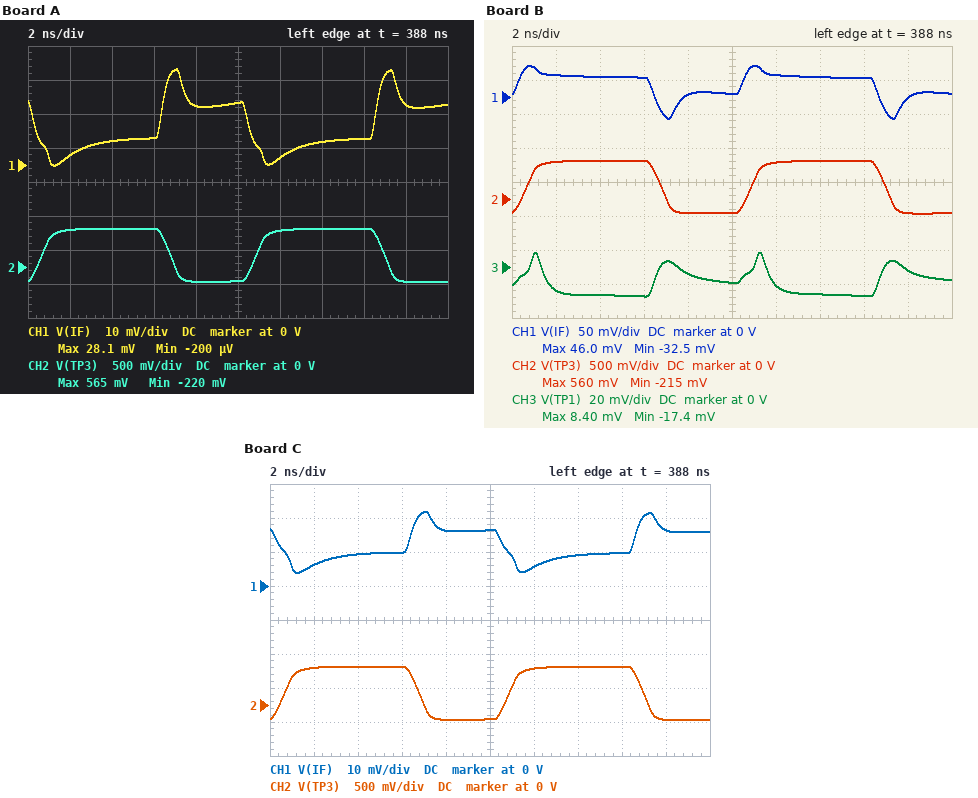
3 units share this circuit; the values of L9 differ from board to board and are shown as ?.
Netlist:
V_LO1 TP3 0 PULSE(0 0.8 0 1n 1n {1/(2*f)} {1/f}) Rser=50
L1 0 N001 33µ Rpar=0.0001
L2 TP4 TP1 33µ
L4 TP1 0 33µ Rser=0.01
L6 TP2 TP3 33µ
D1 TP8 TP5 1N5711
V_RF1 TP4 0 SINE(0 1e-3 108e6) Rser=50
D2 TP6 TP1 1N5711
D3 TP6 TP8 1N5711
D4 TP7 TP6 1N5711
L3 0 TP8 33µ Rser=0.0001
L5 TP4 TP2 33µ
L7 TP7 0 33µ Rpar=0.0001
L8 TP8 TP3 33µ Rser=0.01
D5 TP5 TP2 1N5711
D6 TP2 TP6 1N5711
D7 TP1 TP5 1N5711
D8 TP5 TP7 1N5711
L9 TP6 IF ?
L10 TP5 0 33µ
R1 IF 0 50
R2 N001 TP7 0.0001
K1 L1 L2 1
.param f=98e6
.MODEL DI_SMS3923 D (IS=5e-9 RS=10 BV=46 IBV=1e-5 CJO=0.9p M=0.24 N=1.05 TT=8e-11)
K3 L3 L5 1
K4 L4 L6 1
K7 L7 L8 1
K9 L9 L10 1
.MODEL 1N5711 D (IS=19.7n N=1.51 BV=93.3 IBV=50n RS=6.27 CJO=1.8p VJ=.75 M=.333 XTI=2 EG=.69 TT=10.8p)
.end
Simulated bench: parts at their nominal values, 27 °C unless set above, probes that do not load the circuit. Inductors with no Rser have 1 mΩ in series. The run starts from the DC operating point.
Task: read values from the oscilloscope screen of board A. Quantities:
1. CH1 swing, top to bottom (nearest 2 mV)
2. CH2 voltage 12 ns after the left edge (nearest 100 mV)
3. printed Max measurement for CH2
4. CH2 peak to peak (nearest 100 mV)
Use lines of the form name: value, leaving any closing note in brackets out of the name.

CH1 swing, top to bottom: 28 mV
CH2 voltage 12 ns after the left edge: 500 mV
printed Max measurement for CH2: 565 mV
CH2 peak to peak: 800 mV
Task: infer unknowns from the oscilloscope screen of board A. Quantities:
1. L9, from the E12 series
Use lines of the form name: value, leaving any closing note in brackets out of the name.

L9, from the E12 series: 47 µH
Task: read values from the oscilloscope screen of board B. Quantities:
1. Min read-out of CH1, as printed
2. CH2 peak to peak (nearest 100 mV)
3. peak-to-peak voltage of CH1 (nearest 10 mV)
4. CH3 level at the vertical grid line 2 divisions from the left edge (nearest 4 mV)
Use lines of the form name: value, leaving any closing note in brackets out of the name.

Min read-out of CH1, as printed: -32.5 mV
CH2 peak to peak: 800 mV
peak-to-peak voltage of CH1: 80 mV
CH3 level at the vertical grid line 2 divisions from the left edge: -16 mV
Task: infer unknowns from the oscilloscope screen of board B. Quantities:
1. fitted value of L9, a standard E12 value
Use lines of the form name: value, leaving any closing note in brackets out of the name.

fitted value of L9, a standard E12 value: 10 µH
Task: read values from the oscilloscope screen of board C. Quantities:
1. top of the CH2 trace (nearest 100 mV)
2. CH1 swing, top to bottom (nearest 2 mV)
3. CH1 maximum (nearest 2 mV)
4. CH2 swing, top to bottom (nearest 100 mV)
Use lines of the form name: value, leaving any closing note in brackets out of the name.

top of the CH2 trace: 600 mV
CH1 swing, top to bottom: 18 mV
CH1 maximum: 22 mV
CH2 swing, top to bottom: 800 mV
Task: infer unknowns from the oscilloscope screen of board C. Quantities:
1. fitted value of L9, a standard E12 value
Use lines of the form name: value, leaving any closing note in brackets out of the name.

fitted value of L9, a standard E12 value: 39 µH
